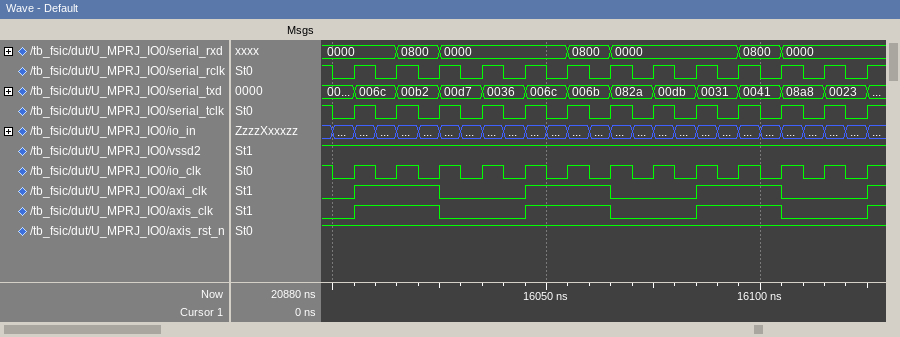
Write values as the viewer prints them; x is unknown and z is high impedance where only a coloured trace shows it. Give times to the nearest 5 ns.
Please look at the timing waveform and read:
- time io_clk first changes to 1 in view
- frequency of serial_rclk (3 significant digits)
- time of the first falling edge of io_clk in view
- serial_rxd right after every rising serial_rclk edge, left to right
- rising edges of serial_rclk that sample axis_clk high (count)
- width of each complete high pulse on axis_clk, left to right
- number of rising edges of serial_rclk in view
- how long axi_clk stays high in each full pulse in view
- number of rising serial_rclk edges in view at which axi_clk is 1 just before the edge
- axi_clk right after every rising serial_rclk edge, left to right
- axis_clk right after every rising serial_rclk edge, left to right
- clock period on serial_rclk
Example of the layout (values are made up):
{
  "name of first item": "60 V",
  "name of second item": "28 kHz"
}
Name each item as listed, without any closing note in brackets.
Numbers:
{
  "time io_clk first changes to 1 in view": "16005 ns",
  "frequency of serial_rclk": "100 MHz",
  "time of the first falling edge of io_clk in view": "16000 ns",
  "serial_rxd right after every rising serial_rclk edge, left to right": "0000, 0800, 0000, 0000, 0000, 0800, 0000, 0000, 0000, 0800, 0000, 0000, 0000",
  "rising edges of serial_rclk that sample axis_clk high": "6",
  "width of each complete high pulse on axis_clk, left to right": "20 ns, 20 ns, 20 ns",
  "number of rising edges of serial_rclk in view": "13",
  "how long axi_clk stays high in each full pulse in view": "20 ns, 20 ns, 20 ns",
  "number of rising serial_rclk edges in view at which axi_clk is 1 just before the edge": "6",
  "axi_clk right after every rising serial_rclk edge, left to right": "1 1 0 0 1 1 0 0 1 1 0 0 1",
  "axis_clk right after every rising serial_rclk edge, left to right": "1 1 0 0 1 1 0 0 1 1 0 0 1",
  "clock period on serial_rclk": "10 ns"
}
